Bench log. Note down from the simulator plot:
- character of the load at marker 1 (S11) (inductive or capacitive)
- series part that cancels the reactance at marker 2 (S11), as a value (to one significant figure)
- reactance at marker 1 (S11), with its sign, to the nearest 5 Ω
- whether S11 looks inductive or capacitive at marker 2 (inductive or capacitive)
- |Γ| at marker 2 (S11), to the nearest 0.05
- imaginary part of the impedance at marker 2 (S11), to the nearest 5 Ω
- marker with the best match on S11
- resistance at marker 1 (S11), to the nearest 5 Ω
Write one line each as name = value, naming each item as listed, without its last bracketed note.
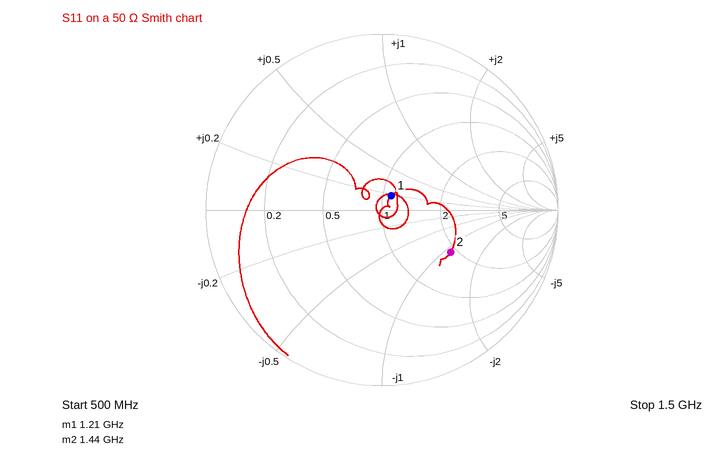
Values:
character of the load at marker 1 (S11) = inductive
series part that cancels the reactance at marker 2 (S11), as a value = 6 nH
reactance at marker 1 (S11), with its sign, to the nearest 5 Ω = +10 Ω
whether S11 looks inductive or capacitive at marker 2 = capacitive
|Γ| at marker 2 (S11), to the nearest 0.05 = 0.45
imaginary part of the impedance at marker 2 (S11), to the nearest 5 Ω = -55 Ω
marker with the best match on S11 = marker 1
resistance at marker 1 (S11), to the nearest 5 Ω = 55 Ω
